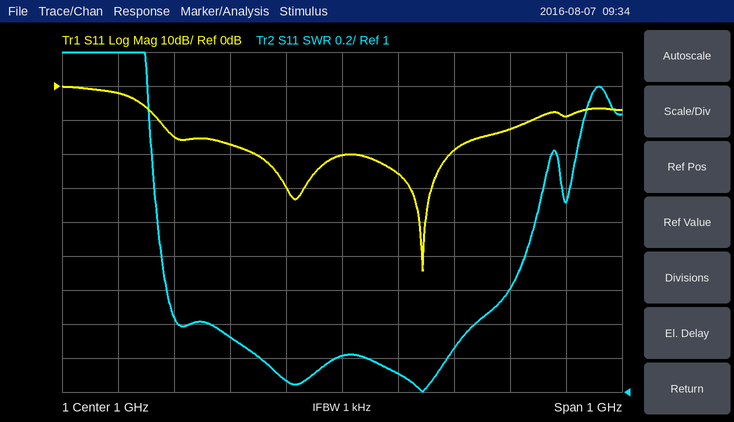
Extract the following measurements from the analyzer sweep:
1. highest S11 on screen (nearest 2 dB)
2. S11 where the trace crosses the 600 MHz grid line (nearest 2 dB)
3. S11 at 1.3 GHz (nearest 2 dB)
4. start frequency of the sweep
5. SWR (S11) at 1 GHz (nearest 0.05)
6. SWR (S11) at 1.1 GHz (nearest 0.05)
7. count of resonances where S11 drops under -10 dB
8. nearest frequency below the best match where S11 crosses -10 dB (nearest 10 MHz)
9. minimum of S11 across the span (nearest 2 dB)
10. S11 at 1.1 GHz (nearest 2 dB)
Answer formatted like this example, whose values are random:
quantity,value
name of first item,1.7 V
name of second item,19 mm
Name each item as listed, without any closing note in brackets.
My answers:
quantity,value
highest S11 on screen,0 dB
S11 where the trace crosses the 600 MHz grid line,-2 dB
S11 at 1.3 GHz,-12 dB
start frequency of the sweep,500 MHz
SWR (S11) at 1 GHz,1.20
SWR (S11) at 1.1 GHz,1.10
count of resonances where S11 drops under -10 dB,2
nearest frequency below the best match where S11 crosses -10 dB,670 MHz
minimum of S11 across the span,-54 dB
S11 at 1.1 GHz,-26 dB
